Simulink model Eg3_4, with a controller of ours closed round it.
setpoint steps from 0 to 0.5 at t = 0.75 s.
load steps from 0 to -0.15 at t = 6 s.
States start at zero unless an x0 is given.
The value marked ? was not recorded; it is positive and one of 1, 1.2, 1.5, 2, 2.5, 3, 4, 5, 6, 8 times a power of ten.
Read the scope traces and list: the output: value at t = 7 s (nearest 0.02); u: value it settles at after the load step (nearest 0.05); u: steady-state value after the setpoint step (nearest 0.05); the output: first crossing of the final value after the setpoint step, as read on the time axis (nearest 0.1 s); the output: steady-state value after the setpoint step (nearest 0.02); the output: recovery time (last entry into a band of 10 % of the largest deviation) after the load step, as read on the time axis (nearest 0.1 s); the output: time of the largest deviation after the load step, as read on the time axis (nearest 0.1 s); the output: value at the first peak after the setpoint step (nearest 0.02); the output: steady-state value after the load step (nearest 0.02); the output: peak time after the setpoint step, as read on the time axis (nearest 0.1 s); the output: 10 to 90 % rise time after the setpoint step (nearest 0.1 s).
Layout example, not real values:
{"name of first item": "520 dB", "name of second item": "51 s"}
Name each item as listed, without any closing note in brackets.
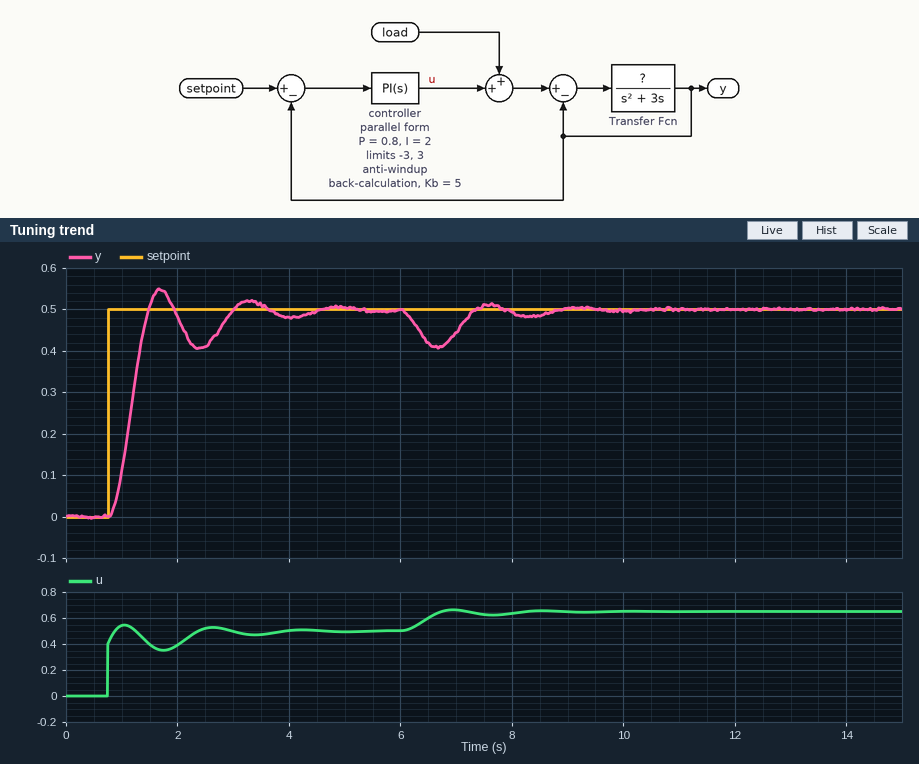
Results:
{"the output: value at t = 7 s": "0.44", "u: value it settles at after the load step": "0.65", "u: steady-state value after the setpoint step": "0.50", "the output: first crossing of the final value after the setpoint step, as read on the time axis": "1.5 s", "the output: steady-state value after the setpoint step": "0.50", "the output: recovery time (last entry into a band of 10 % of the largest deviation) after the load step, as read on the time axis": "8.7 s", "the output: time of the largest deviation after the load step, as read on the time axis": "6.7 s", "the output: value at the first peak after the setpoint step": "0.54", "the output: steady-state value after the load step": "0.50", "the output: peak time after the setpoint step, as read on the time axis": "1.7 s", "the output: 10 to 90 % rise time after the setpoint step": "0.5 s"}
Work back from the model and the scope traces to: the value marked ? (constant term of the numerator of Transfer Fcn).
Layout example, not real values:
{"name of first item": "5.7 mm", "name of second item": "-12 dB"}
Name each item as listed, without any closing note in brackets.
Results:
{"the value marked ?": "10"}
